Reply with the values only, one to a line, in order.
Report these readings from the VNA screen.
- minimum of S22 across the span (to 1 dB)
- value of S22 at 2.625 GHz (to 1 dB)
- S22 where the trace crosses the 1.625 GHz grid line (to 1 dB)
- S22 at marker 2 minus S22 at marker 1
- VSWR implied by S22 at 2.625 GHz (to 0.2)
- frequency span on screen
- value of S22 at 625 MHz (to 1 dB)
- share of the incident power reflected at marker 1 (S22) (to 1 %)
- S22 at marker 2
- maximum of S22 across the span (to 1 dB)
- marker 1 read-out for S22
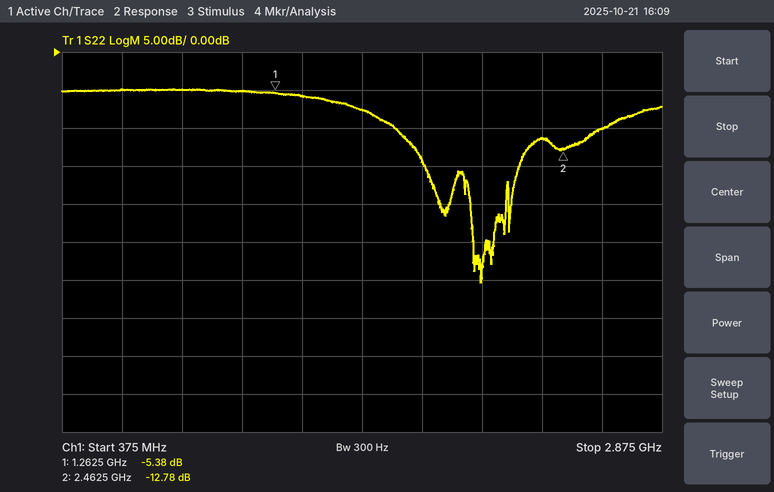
-30 dB
-10 dB
-8 dB
-7.40 dB
2.0
2.5 GHz
-5 dB
29 %
-12.78 dB
-5 dB
-5.38 dB
